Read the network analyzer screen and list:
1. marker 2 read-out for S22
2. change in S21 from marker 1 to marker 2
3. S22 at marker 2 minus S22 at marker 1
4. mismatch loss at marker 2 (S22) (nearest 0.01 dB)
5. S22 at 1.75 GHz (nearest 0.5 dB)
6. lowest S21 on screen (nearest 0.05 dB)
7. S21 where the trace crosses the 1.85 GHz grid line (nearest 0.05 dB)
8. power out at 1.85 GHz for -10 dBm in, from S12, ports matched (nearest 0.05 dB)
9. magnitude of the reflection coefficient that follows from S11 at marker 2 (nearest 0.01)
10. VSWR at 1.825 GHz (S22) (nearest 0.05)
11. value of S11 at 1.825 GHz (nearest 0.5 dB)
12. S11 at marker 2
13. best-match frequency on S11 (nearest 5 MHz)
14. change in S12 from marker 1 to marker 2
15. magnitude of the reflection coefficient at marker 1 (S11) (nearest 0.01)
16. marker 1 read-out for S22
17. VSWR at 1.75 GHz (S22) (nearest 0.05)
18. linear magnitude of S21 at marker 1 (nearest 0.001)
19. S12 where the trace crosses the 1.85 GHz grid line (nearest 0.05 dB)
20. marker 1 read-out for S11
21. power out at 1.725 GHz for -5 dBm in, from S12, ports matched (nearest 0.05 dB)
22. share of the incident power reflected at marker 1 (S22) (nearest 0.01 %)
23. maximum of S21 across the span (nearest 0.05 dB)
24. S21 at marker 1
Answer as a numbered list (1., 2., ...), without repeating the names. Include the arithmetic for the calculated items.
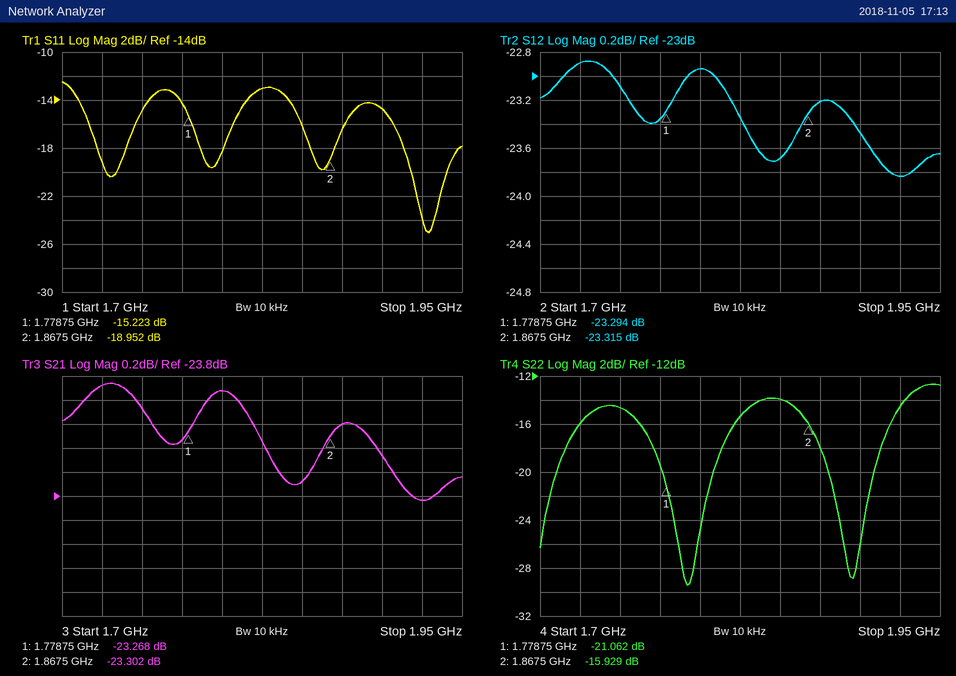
1. -15.929 dB
2. -23.302 − (-23.268) = -0.034 dB
3. -15.929 − (-21.062) = 5.133 dB
4. −10 log10(1 − 10^(-15.929/10)) ≈ 0.11 dB
5. -14.5 dB
6. -23.85 dB
7. -23.70 dB
8. -10 dBm + (-23.70 dB) = -33.70 dBm
9. 10^(-18.952/20) ≈ 0.11
10. |Γ| = 10^(-15.5/20) = 0.1679; VSWR = (1 + 0.1679)/(1 − 0.1679) ≈ 1.40
11. -13.0 dB
12. -18.952 dB
13. 1.930 GHz
14. -23.315 − (-23.294) = -0.021 dB
15. 10^(-15.223/20) ≈ 0.17
16. -21.062 dB
17. |Γ| = 10^(-14.5/20) = 0.1884; VSWR = (1 + 0.1884)/(1 − 0.1884) ≈ 1.46, so 1.45 to the nearest 0.05
18. 10^(-23.268/20) ≈ 0.069
19. -23.70 dB
20. -15.223 dB
21. -5 dBm + (-22.90 dB) = -27.90 dBm
22. 10^(-21.062/10) ≈ 0.78 %
23. -22.85 dB
24. -23.268 dB
